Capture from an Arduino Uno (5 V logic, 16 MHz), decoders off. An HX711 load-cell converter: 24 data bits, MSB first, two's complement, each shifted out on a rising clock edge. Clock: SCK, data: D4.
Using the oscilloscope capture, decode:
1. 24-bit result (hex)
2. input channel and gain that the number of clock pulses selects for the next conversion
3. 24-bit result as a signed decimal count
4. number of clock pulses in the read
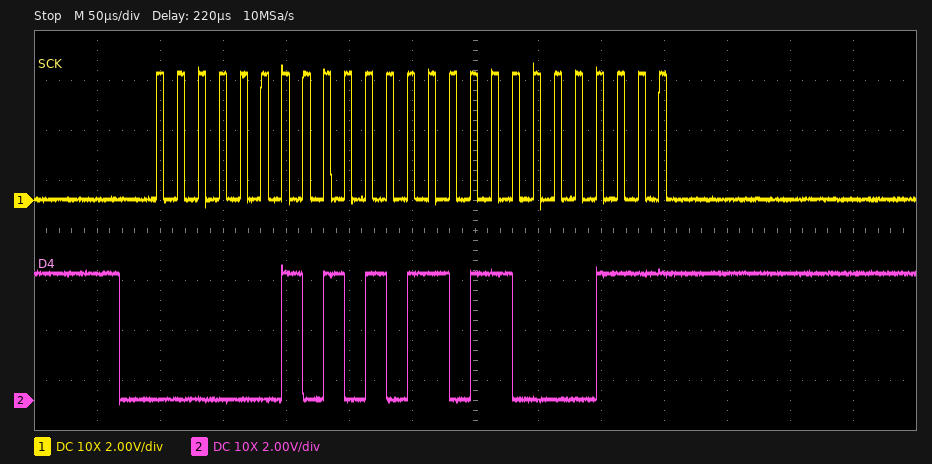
0x02AD87
channel A, gain 128
175495
25
